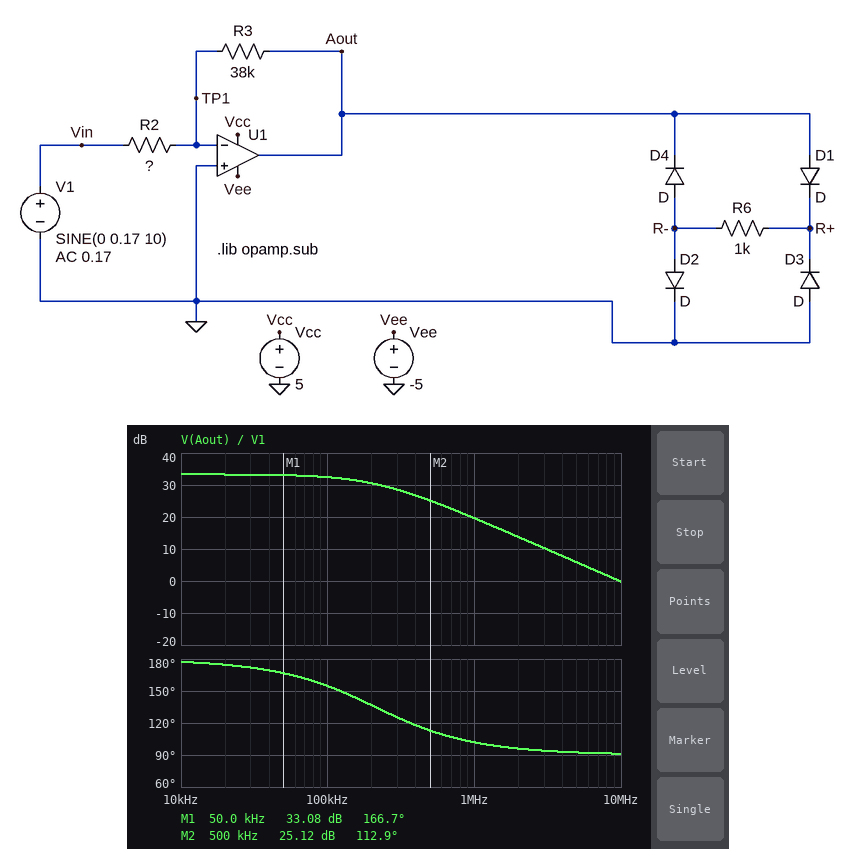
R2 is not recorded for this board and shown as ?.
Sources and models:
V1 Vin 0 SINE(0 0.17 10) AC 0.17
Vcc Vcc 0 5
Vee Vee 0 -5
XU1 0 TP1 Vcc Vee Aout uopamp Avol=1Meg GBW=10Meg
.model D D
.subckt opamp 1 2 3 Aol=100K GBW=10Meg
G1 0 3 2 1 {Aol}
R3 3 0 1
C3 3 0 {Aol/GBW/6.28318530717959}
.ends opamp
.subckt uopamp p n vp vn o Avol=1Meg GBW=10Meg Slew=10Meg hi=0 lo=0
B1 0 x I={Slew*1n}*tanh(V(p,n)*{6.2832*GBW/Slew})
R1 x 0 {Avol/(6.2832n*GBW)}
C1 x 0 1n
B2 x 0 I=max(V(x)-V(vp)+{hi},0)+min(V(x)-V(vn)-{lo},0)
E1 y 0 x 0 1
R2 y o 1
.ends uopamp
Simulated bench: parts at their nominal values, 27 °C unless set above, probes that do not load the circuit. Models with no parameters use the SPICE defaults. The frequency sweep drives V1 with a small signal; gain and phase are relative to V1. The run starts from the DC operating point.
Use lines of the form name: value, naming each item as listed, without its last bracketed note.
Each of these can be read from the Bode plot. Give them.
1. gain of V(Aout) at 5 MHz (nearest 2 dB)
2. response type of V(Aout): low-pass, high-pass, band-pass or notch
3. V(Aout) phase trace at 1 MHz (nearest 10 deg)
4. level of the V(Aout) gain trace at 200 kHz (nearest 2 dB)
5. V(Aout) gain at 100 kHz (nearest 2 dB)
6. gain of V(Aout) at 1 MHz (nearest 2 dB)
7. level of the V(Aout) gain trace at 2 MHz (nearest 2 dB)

gain of V(Aout) at 5 MHz: 6 dB
response type of V(Aout): low-pass, high-pass, band-pass or notch: low-pass
V(Aout) phase trace at 1 MHz: 100 deg
level of the V(Aout) gain trace at 200 kHz: 30 dB
V(Aout) gain at 100 kHz: 32 dB
gain of V(Aout) at 1 MHz: 20 dB
level of the V(Aout) gain trace at 2 MHz: 14 dB
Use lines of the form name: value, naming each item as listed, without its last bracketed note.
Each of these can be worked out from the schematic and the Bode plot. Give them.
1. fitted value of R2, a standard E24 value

fitted value of R2, a standard E24 value: 820 Ω
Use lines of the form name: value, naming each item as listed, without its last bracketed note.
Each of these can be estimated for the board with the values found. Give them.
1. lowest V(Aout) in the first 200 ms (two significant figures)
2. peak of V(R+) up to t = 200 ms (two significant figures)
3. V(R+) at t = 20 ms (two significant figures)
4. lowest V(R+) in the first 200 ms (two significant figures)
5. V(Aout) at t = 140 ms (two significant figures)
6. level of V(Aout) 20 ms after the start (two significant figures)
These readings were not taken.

lowest V(Aout) in the first 200 ms: -5.0 V
peak of V(R+) up to t = 200 ms: 4.3 V
V(R+) at t = 20 ms: -690 mV
lowest V(R+) in the first 200 ms: -690 mV
V(Aout) at t = 140 ms: -4.6 V
level of V(Aout) 20 ms after the start: -5.0 V
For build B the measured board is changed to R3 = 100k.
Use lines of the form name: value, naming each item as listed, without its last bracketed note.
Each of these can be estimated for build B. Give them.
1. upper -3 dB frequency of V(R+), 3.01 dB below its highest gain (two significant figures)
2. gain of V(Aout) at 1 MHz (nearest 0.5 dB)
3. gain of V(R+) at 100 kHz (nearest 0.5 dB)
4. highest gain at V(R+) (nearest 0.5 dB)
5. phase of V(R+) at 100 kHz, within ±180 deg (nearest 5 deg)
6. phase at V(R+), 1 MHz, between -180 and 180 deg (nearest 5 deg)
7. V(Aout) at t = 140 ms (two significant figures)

upper -3 dB frequency of V(R+), 3.01 dB below its highest gain: 81 kHz
gain of V(Aout) at 1 MHz: 20.0 dB
gain of V(R+) at 100 kHz: 31.5 dB
highest gain at V(R+): 35.5 dB
phase of V(R+) at 100 kHz, within ±180 deg: 130 deg
phase at V(R+), 1 MHz, between -180 and 180 deg: 95 deg
V(Aout) at t = 140 ms: -5.0 V
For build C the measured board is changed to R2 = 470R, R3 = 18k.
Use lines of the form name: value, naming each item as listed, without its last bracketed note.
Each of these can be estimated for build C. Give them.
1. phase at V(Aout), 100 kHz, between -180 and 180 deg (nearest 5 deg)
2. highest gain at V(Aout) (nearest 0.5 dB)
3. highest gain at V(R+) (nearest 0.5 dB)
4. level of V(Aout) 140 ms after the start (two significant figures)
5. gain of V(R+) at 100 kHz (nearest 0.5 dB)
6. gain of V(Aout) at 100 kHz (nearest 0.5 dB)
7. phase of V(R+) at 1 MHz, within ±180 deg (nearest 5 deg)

phase at V(Aout), 100 kHz, between -180 and 180 deg: 160 deg
highest gain at V(Aout): 31.5 dB
highest gain at V(R+): 25.5 dB
level of V(Aout) 140 ms after the start: -3.8 V
gain of V(R+) at 100 kHz: 25.0 dB
gain of V(Aout) at 100 kHz: 31.0 dB
phase of V(R+) at 1 MHz, within ±180 deg: 105 deg
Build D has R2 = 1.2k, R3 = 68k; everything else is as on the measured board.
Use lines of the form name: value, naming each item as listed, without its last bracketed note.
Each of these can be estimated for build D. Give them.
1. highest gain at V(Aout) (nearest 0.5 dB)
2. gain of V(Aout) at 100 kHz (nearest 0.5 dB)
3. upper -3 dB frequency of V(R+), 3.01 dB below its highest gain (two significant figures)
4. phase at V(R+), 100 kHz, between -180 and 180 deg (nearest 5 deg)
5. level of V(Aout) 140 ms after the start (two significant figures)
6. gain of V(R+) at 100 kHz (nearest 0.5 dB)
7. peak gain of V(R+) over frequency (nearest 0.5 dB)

highest gain at V(Aout): 35.0 dB
gain of V(Aout) at 100 kHz: 34.0 dB
upper -3 dB frequency of V(R+), 3.01 dB below its highest gain: 170 kHz
phase at V(R+), 100 kHz, between -180 and 180 deg: 150 deg
level of V(Aout) 140 ms after the start: -5.0 V
gain of V(R+) at 100 kHz: 28.0 dB
peak gain of V(R+) over frequency: 29.0 dB
